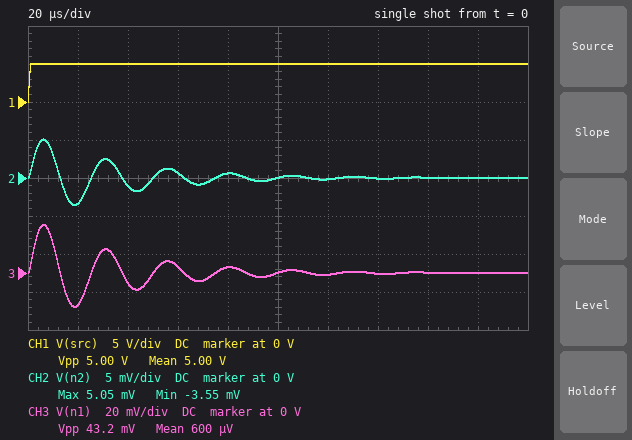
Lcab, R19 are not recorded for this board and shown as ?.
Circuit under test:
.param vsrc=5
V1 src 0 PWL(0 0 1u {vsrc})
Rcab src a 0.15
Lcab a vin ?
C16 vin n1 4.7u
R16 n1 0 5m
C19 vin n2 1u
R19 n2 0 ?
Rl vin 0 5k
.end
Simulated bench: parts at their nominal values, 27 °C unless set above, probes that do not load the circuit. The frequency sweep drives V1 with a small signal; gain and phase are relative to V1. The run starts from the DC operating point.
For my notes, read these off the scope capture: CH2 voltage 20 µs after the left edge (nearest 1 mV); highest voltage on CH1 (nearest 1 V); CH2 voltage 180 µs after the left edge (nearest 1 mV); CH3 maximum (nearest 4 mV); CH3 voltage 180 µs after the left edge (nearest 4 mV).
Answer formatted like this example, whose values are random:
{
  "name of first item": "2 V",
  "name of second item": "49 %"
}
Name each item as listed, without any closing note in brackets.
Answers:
{
  "CH2 voltage 20 µs after the left edge": "-3 mV",
  "highest voltage on CH1": "5 V",
  "CH2 voltage 180 µs after the left edge": "0 V",
  "CH3 maximum": "24 mV",
  "CH3 voltage 180 µs after the left edge": "0 V"
}
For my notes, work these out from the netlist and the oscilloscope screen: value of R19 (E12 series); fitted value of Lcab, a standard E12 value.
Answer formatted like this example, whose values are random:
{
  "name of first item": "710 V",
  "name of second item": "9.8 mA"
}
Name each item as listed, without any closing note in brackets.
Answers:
{
  "value of R19": "4.7 mΩ",
  "fitted value of Lcab, a standard E12 value": "2.7 µH"
}
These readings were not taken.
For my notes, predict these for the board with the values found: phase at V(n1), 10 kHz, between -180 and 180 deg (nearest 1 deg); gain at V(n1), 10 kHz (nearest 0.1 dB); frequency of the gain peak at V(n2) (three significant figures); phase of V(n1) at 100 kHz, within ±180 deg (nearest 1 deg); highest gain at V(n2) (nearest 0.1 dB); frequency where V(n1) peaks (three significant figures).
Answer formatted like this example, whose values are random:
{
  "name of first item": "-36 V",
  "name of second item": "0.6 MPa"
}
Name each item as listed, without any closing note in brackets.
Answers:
{
  "phase at V(n1), 10 kHz, between -180 and 180 deg": "87 deg",
  "gain at V(n1), 10 kHz": "-56.1 dB",
  "frequency of the gain peak at V(n2)": "40.6 kHz",
  "phase of V(n1) at 100 kHz, within ±180 deg": "-84 deg",
  "highest gain at V(n2)": "-45.4 dB",
  "frequency where V(n1) peaks": "40.6 kHz"
}
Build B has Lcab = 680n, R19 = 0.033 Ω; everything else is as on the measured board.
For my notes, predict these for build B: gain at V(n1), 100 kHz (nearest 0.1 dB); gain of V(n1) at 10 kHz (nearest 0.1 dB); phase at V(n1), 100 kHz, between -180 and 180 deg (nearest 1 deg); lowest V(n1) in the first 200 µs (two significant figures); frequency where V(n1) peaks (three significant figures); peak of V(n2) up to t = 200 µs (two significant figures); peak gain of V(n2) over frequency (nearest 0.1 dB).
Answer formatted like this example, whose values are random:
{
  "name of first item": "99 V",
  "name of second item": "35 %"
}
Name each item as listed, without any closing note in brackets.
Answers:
{
  "gain at V(n1), 100 kHz": "-34.3 dB",
  "gain of V(n1) at 10 kHz": "-56.5 dB",
  "phase at V(n1), 100 kHz, between -180 and 180 deg": "-44 deg",
  "lowest V(n1) in the first 200 µs": "-21 mV",
  "frequency where V(n1) peaks": "80.8 kHz",
  "peak of V(n2) up to t = 200 µs": "61 mV",
  "peak gain of V(n2) over frequency": "-28.5 dB"
}
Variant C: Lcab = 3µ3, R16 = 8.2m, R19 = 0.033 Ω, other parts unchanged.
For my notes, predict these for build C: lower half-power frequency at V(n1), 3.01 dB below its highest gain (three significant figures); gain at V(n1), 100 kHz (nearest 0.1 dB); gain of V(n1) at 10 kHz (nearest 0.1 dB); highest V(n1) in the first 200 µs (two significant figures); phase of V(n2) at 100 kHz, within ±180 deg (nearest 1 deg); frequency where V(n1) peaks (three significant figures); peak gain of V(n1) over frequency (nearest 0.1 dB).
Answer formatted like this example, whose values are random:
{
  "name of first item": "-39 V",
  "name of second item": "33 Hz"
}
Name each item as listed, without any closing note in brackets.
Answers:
{
  "lower half-power frequency at V(n1), 3.01 dB below its highest gain": "33.1 kHz",
  "gain at V(n1), 100 kHz": "-48.5 dB",
  "gain of V(n1) at 10 kHz": "-51.7 dB",
  "highest V(n1) in the first 200 µs": "38 mV",
  "phase of V(n2) at 100 kHz, within ±180 deg": "-85 deg",
  "frequency where V(n1) peaks": "36.7 kHz",
  "peak gain of V(n1) over frequency": "-27.3 dB"
}
